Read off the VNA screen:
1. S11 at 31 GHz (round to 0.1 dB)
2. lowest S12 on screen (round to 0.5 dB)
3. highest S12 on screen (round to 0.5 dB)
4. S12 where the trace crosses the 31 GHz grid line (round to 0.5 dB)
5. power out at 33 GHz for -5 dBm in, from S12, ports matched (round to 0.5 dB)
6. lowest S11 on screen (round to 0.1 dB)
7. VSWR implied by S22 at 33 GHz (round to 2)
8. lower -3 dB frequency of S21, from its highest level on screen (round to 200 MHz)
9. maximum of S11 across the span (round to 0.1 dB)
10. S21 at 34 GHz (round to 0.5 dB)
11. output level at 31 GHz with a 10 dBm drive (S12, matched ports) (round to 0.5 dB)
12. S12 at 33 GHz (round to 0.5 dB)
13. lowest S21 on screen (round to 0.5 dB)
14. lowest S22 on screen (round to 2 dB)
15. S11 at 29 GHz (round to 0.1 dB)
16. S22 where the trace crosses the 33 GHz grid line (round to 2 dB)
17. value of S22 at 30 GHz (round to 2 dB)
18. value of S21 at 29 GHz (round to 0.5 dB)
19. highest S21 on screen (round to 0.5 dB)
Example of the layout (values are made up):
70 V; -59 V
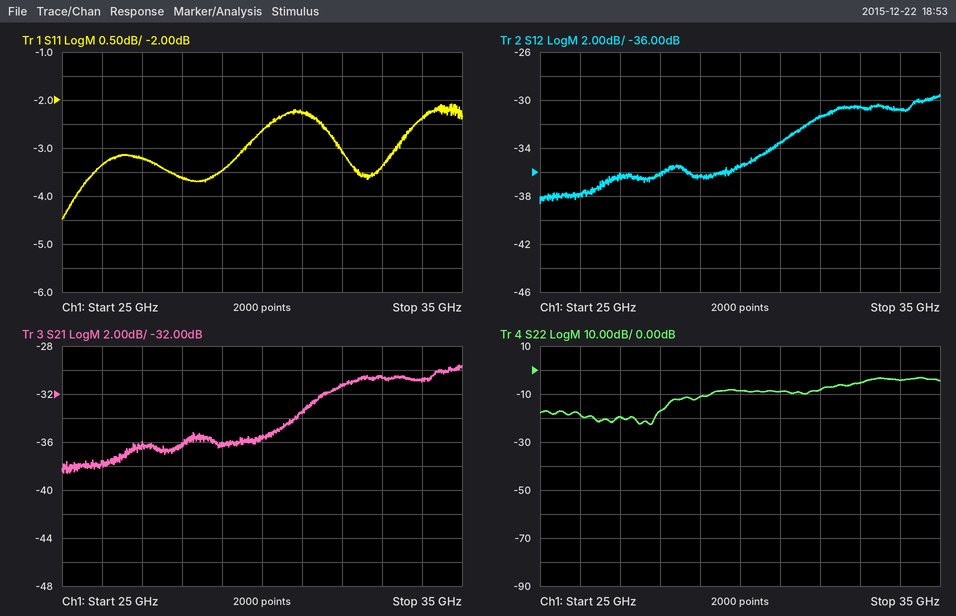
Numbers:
-2.3 dB; -38.5 dB; -29.5 dB; -33.5 dB; -35.5 dBm; -4.5 dB; 4; 31.4 GHz; -2.1 dB; -31.0 dB; -23.5 dBm; -30.5 dB; -38.5 dB; -22 dB; -3.5 dB; -6 dB; -8 dB; -36.0 dB; -29.5 dB
